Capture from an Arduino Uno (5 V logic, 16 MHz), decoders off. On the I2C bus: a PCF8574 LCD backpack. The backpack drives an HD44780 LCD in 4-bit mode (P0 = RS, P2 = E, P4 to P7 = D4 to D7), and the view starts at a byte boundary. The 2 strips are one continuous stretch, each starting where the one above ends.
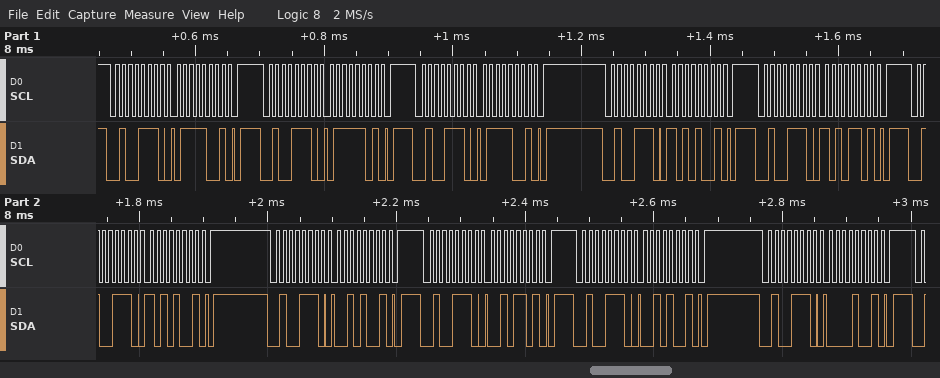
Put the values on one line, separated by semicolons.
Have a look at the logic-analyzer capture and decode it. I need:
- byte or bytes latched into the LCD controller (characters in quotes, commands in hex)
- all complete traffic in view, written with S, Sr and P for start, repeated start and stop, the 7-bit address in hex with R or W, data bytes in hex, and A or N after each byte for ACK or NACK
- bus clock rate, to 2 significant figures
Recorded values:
'z'; S 27W A 79 A P S 27W A 7D A P S 27W A 79 A P S 27W A A9 A P S 27W A AD A P S 27W A A9 A P S 27W A 29 A P S 27W A 2D A P S 27W A 29 A P S 27W A 09 A P; 100 kHz
